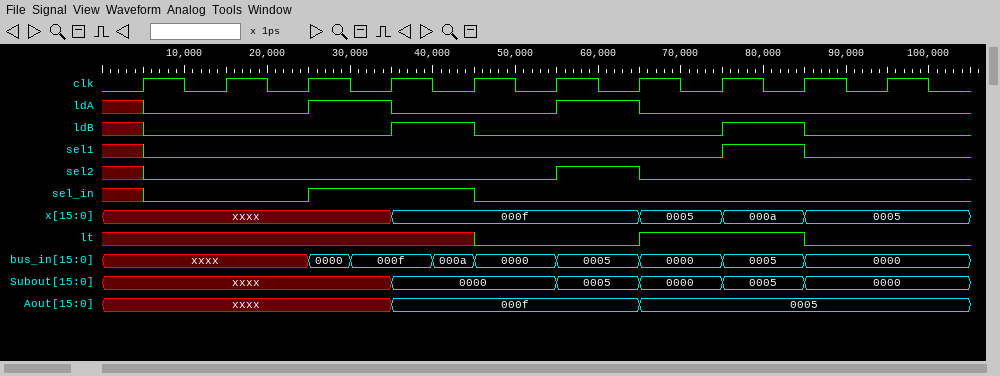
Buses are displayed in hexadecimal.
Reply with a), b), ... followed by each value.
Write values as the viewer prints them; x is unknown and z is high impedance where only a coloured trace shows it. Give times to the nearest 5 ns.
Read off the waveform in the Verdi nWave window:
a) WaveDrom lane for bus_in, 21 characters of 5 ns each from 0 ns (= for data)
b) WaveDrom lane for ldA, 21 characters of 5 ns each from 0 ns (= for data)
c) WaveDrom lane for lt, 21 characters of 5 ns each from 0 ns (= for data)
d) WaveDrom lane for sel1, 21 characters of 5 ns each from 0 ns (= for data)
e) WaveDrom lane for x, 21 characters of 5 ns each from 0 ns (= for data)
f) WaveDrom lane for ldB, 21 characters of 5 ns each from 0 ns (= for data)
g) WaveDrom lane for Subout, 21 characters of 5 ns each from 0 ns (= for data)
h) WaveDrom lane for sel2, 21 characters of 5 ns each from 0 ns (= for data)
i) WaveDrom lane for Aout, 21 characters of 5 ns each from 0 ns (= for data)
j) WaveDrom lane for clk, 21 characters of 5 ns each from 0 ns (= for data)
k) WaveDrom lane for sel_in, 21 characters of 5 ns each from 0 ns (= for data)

a) {name: 'bus_in', wave: 'x....==.==.=.=.=.=...', data: '0000 000f 000a 0000 0005 0000 0005 0000'}
b) {name: 'ldA', wave: 'x0...1.0...1.0.......'}
c) {name: 'lt', wave: 'x........0...1...0...'}
d) {name: 'sel1', wave: 'x0.............1.0...'}
e) {name: 'x', wave: 'x......=.....=.=.=...', data: '000f 0005 000a 0005'}
f) {name: 'ldB', wave: 'x0.....1.0.....1.0...'}
g) {name: 'Subout', wave: 'x......=...=.=.=.=...', data: '0000 0005 0000 0005 0000'}
h) {name: 'sel2', wave: 'x0.........1.0.......'}
i) {name: 'Aout', wave: 'x......=.....=.......', data: '000f 0005'}
j) {name: 'clk', wave: '010101010101010101010'}
k) {name: 'sel_in', wave: 'x0...1...0...........'}
